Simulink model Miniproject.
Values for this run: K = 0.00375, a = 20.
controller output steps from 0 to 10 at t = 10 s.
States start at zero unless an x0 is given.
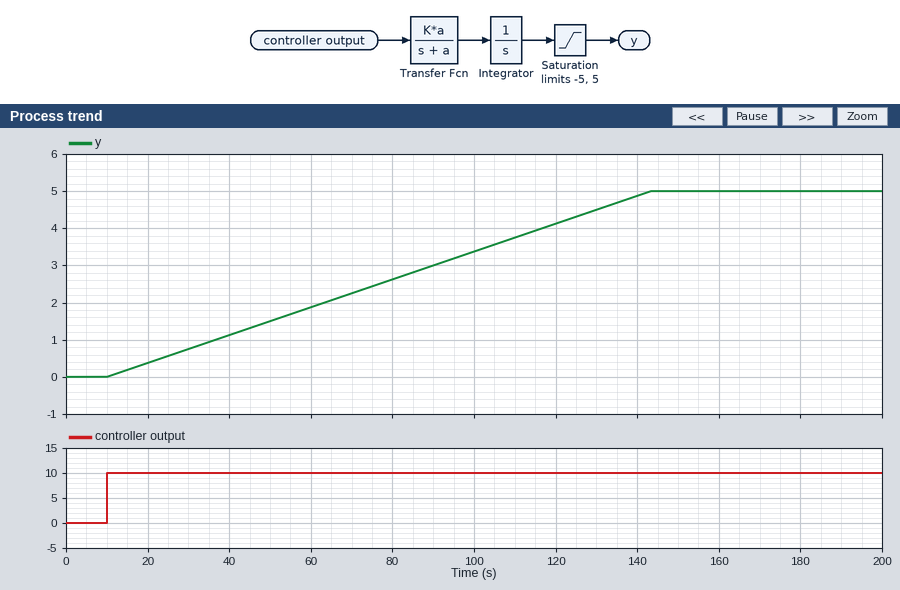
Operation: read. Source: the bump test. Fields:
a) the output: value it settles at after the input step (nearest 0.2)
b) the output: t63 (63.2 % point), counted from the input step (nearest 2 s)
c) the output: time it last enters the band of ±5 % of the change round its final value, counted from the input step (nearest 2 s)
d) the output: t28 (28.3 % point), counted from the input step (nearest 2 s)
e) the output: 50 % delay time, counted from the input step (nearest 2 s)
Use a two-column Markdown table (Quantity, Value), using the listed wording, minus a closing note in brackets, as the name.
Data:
| Quantity | Value |
|---|---|
| the output: value it settles at after the input step | 5.0 |
| the output: t63 (63.2 % point), counted from the input step | 84 s |
| the output: time it last enters the band of ±5 % of the change round its final value, counted from the input step | 126 s |
| the output: t28 (28.3 % point), counted from the input step | 38 s |
| the output: 50 % delay time, counted from the input step | 66 s |
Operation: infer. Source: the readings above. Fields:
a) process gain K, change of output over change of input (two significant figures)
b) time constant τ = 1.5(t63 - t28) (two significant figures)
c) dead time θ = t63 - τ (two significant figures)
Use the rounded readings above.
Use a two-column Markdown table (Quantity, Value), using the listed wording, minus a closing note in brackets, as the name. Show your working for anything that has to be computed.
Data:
| Quantity | Value |
|---|---|
| process gain K, change of output over change of input | (5 - 0) / 10 = 0.50 |
| time constant τ = 1.5(t63 - t28) | 1.5 × (84 - 38) = 69 s |
| dead time θ = t63 - τ | 84 - 69 = 15 s |
